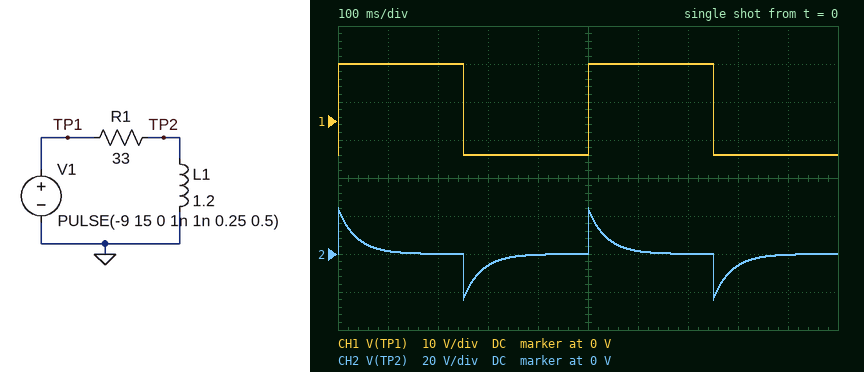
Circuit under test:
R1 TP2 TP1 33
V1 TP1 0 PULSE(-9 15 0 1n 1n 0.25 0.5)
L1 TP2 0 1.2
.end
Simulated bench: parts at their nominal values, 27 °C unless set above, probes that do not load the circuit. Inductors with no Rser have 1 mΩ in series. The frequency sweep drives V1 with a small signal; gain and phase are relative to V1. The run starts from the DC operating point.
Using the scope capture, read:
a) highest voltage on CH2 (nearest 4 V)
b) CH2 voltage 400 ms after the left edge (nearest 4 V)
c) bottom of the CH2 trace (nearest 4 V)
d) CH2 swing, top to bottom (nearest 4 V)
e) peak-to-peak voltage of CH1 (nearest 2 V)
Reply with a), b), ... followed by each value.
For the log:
a) 24 V
b) 0 V
c) -24 V
d) 48 V
e) 24 V
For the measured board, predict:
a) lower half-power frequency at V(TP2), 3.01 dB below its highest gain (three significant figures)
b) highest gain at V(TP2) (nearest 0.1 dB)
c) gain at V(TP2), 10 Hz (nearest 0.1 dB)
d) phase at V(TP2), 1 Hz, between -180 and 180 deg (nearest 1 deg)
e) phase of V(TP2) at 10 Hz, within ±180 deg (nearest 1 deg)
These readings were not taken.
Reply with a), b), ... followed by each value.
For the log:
a) 4.38 Hz
b) 0 dB
c) -0.8 dB
d) 77 deg
e) 24 deg
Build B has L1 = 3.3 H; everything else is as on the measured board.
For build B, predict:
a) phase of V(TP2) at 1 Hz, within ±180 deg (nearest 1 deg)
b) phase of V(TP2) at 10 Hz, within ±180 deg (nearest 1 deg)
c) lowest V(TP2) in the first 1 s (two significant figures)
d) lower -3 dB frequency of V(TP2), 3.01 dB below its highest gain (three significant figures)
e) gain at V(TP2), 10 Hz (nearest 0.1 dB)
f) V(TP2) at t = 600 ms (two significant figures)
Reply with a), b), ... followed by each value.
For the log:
a) 58 deg
b) 9 deg
c) -22 V
d) 1.59 Hz
e) -0.1 dB
f) 8.2 V
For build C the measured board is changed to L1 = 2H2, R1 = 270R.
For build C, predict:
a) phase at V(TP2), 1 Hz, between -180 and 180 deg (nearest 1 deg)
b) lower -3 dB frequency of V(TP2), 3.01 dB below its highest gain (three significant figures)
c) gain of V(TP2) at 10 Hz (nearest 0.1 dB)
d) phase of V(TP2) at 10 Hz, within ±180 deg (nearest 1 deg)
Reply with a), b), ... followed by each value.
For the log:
a) 87 deg
b) 19.5 Hz
c) -6.8 dB
d) 63 deg
